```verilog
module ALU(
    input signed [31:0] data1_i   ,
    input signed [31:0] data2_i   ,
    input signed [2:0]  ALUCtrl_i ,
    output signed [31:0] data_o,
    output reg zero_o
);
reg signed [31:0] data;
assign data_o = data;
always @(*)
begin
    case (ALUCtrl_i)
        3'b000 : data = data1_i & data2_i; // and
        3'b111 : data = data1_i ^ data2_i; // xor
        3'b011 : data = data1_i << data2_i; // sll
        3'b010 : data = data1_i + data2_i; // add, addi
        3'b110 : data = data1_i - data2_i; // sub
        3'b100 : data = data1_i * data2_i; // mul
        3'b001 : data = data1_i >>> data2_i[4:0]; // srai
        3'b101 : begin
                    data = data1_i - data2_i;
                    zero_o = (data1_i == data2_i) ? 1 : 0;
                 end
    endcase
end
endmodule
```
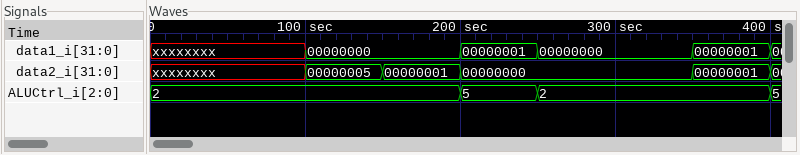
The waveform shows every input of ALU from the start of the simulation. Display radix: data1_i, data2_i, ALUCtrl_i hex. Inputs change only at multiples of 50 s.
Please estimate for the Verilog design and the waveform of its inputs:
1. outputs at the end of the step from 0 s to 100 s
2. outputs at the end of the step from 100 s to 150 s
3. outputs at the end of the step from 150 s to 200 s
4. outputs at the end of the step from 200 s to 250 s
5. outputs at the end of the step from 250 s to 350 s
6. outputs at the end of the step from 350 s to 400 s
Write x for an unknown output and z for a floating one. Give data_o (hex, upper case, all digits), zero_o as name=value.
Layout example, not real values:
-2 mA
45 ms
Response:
data_o=x, zero_o=x
data_o=00000005, zero_o=x
data_o=00000001, zero_o=x
data_o=00000001, zero_o=0
data_o=00000000, zero_o=0
data_o=00000002, zero_o=0
